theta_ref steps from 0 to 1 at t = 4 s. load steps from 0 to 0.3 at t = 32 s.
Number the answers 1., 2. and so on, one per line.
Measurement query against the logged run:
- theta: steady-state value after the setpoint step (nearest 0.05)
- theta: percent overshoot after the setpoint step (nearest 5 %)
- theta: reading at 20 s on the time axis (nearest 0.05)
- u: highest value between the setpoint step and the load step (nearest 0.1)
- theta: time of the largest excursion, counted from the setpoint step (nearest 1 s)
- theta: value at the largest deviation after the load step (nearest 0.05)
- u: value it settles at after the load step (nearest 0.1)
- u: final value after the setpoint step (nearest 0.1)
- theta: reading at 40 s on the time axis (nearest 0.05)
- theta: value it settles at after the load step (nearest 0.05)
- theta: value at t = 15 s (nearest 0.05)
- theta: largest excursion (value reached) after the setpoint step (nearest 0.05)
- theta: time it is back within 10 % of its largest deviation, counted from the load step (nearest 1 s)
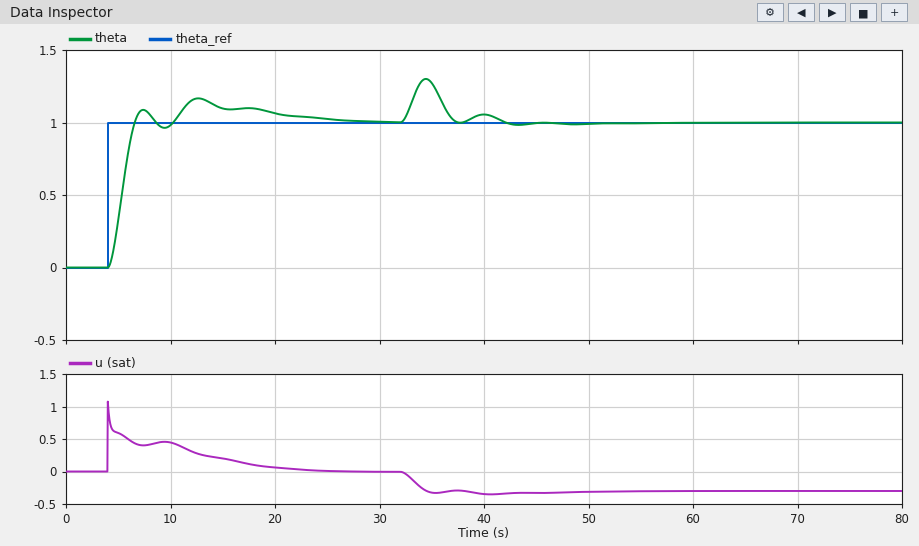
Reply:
1. 1.00
2. 15 %
3. 1.05
4. 1.1
5. 9 s
6. 1.30
7. -0.3
8. 0.0
9. 1.05
10. 1.00
11. 1.10
12. 1.15
13. 9 s
